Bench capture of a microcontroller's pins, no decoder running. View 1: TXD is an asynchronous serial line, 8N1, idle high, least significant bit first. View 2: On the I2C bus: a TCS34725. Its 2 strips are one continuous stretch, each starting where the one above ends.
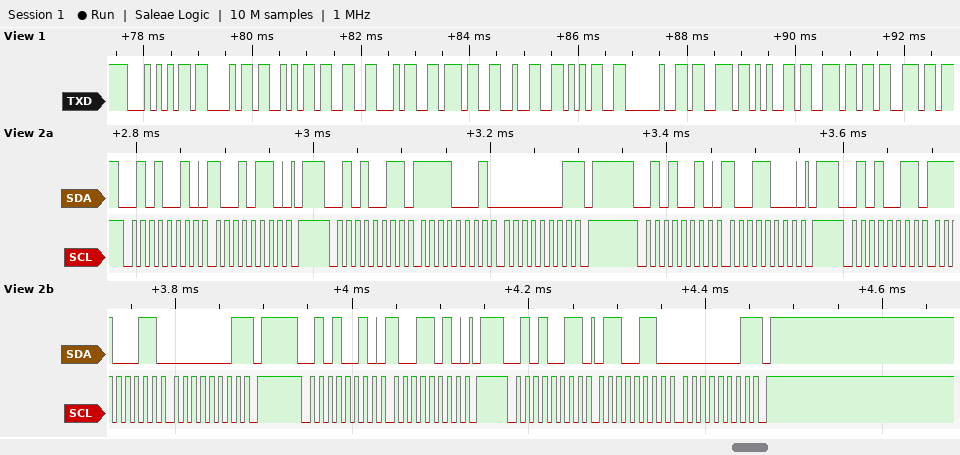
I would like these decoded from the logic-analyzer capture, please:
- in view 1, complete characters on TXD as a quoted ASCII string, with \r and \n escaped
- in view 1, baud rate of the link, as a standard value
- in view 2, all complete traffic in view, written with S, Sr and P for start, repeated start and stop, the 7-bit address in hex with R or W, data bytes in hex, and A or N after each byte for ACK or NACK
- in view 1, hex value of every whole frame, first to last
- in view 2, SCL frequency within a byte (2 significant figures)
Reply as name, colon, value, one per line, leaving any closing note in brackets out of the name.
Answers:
in view 1, complete characters on TXD as a quoted ASCII string, with \r and \n escaped: "TCS34725 sens"
in view 1, baud rate of the link, as a standard value: 9600 baud
in view 2, all complete traffic in view, written with S, Sr and P for start, repeated start and stop, the 7-bit address in hex with R or W, data bytes in hex, and A or N after each byte for ACK or NACK: S 29W A 96 A P S 29R A F1 A 01 N P S 29W A 98 A P S 29R A E3 A 01 N P S 29W A 9A A P S 29R A 66 A 01 N P
in view 1, hex value of every whole frame, first to last: 54 43 53 33 34 37 32 35 20 73 65 6E 73
in view 2, SCL frequency within a byte: 100 kHz
